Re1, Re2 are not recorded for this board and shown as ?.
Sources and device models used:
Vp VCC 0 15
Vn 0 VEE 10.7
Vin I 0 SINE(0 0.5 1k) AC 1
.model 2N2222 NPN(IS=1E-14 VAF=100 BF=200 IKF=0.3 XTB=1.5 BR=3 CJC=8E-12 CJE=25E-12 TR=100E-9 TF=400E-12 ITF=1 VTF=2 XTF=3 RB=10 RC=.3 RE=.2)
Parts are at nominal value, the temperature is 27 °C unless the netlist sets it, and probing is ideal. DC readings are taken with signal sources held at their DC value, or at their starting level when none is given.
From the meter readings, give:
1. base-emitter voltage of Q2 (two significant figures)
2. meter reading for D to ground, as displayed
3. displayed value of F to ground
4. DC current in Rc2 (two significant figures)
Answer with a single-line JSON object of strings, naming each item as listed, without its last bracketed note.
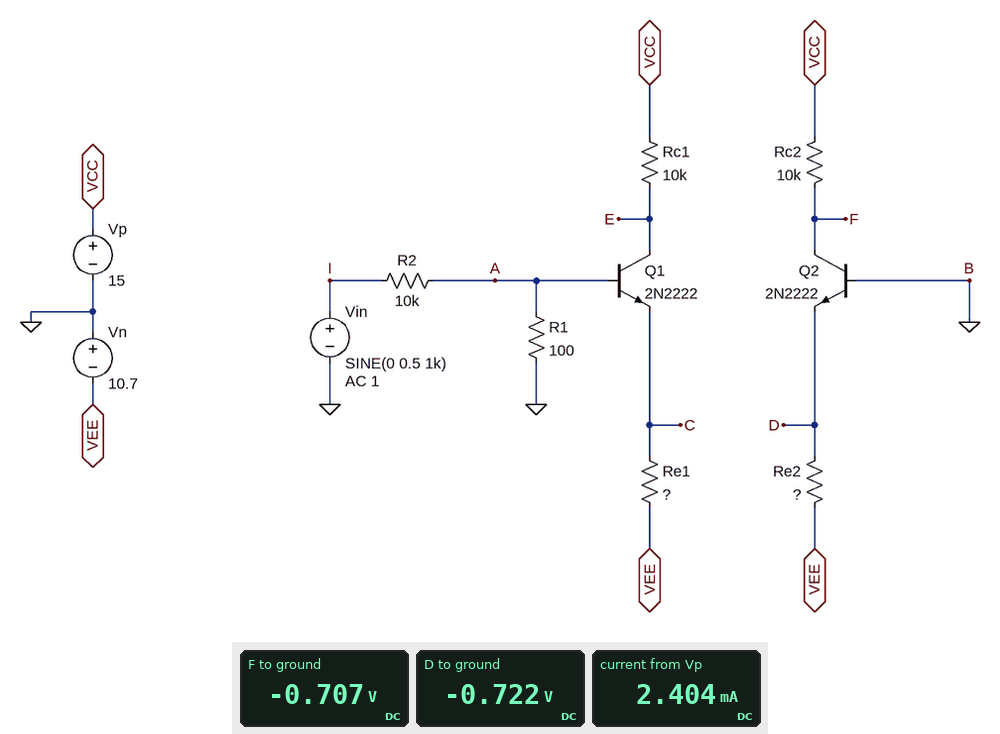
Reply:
{"base-emitter voltage of Q2": "720 mV", "meter reading for D to ground, as displayed": "-0.722 V", "displayed value of F to ground": "-0.707 V", "DC current in Rc2": "1.6 mA"}
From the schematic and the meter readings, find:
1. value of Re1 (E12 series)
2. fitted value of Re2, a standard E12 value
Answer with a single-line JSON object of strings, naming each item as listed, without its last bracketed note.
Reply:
{"value of Re1": "12 kΩ", "fitted value of Re2, a standard E12 value": "3.3 kΩ"}
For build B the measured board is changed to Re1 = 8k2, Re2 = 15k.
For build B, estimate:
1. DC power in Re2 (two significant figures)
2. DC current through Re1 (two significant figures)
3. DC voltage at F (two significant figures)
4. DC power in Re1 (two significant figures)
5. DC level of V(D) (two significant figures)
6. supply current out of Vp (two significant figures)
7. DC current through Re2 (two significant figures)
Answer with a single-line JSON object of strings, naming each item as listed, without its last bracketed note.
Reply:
{"DC power in Re2": "6.7 mW", "DC current through Re1": "1.2 mA", "DC voltage at F": "8.3 V", "DC power in Re1": "12 mW", "DC level of V(D)": "-640 mV", "supply current out of Vp": "1.9 mA", "DC current through Re2": "670 µA"}
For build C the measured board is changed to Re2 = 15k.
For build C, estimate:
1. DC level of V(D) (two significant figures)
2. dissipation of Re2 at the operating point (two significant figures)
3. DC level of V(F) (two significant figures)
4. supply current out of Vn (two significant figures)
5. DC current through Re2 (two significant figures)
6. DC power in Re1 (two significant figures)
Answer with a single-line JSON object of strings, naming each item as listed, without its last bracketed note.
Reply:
{"DC level of V(D)": "-640 mV", "dissipation of Re2 at the operating point": "6.7 mW", "DC level of V(F)": "8.3 V", "supply current out of Vn": "1.5 mA", "DC current through Re2": "670 µA", "DC power in Re1": "8.4 mW"}
